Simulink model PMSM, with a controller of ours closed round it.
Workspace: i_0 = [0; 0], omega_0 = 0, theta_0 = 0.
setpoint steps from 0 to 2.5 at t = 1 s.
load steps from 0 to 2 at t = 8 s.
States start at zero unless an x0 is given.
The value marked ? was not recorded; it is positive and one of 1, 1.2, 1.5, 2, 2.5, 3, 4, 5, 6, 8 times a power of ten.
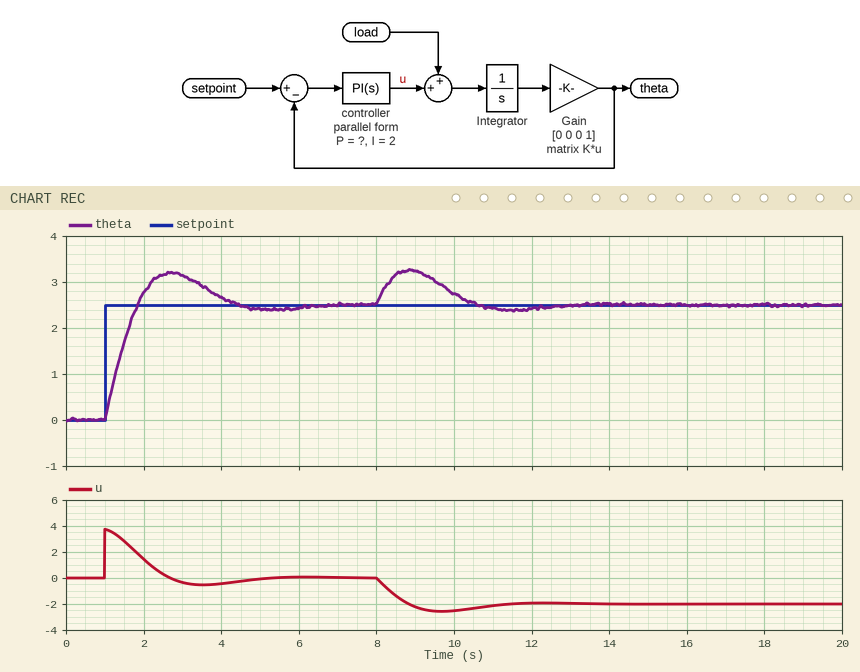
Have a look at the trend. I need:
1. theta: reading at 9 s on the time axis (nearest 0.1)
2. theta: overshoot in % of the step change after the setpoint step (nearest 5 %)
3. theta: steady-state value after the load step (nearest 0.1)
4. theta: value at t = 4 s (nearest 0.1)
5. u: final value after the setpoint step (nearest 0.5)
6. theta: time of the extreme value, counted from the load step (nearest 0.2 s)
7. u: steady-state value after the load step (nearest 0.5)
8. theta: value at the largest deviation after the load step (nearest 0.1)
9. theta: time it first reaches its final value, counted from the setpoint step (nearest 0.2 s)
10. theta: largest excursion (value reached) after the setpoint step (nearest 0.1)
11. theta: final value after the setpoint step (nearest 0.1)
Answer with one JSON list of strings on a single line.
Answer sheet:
["3.2", "30 %", "2.5", "2.7", "0.0", "0.8 s", "-2.0", "3.3", "0.8 s", "3.2", "2.5"]
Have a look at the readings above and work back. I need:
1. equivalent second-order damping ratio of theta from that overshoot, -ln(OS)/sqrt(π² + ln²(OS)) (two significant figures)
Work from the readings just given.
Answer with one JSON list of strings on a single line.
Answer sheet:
["0.36"]
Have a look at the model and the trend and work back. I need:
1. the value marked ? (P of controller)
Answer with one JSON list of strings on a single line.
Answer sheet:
["1.5"]
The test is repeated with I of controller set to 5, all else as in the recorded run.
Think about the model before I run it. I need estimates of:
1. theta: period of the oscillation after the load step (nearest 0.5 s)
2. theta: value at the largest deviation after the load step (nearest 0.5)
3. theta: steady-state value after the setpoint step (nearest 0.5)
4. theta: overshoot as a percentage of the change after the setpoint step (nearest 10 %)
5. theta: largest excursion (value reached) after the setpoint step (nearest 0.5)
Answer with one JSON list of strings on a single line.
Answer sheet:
["3.0 s", "3.0", "2.5", "40 %", "3.5"]
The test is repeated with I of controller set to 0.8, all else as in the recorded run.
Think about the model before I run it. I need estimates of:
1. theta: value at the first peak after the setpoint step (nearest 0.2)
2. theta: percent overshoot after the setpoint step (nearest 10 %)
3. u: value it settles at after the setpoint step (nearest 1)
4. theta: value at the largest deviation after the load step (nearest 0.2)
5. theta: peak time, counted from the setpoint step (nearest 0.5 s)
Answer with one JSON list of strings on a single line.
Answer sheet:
["3.0", "20 %", "0", "3.4", "2.5 s"]
